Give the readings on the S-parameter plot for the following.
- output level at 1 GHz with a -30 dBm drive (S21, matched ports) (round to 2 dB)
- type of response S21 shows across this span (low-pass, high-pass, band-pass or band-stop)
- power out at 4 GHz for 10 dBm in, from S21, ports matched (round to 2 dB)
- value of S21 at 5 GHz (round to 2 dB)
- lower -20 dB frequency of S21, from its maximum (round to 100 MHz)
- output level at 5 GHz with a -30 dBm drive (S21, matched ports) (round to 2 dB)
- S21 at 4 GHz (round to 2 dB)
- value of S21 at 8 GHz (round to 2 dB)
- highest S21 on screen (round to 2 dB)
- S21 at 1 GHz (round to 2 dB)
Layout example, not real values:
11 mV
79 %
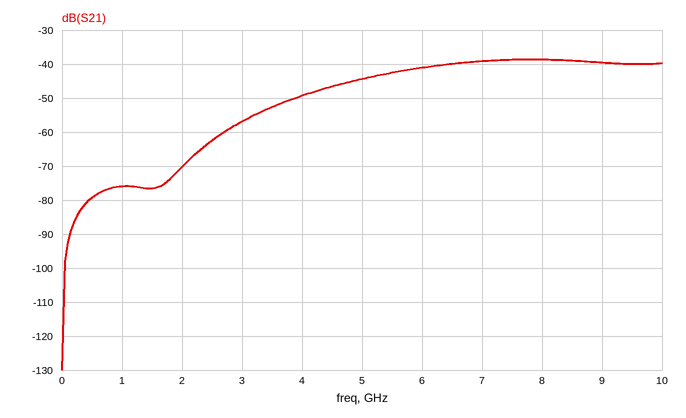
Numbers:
-106 dBm
high-pass
-40 dBm
-44 dB
2.8 GHz
-74 dBm
-50 dB
-38 dB
-38 dB
-76 dB
